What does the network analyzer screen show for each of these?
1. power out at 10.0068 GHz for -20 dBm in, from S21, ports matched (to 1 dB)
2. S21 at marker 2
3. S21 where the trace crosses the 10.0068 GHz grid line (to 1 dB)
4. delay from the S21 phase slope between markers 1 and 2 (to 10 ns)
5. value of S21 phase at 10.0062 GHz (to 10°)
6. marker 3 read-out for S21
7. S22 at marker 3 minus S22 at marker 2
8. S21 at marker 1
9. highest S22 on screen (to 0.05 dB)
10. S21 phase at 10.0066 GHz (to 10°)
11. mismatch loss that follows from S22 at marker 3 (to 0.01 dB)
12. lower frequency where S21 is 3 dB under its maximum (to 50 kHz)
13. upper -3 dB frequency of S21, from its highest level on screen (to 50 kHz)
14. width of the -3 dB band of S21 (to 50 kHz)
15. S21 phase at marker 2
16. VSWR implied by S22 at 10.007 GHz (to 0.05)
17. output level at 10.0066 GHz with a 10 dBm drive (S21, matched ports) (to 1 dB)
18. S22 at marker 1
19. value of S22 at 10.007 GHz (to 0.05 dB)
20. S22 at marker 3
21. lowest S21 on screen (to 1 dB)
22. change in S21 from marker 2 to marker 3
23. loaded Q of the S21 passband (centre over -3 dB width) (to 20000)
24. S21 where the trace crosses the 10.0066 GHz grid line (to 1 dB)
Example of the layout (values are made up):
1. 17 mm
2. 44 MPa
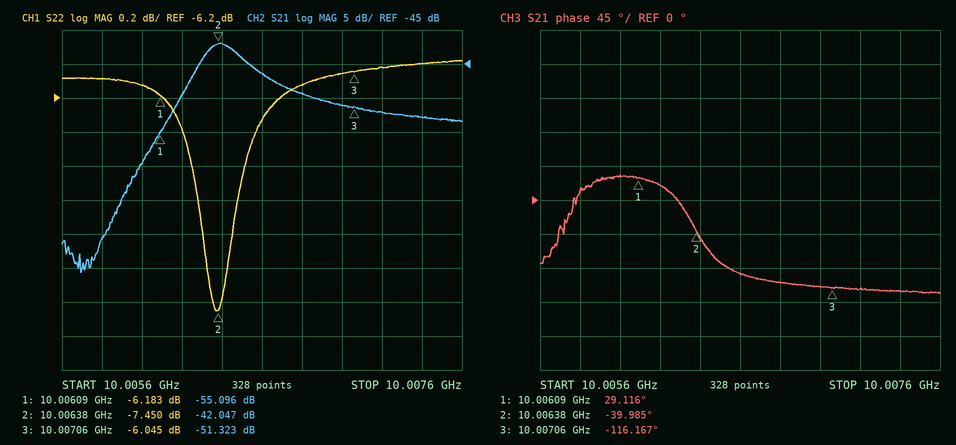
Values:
1. -69 dBm
2. -42.047 dB
3. -49 dB
4. 660 ns
5. 20°
6. -51.323 dB
7. 1.405 dB
8. -55.096 dB
9. -6.00 dB
10. -100°
11. 1.24 dB
12. 10.00630 GHz
13. 10.00655 GHz
14. 250 kHz
15. -39.985°
16. 3.00
17. -36 dBm
18. -6.183 dB
19. -6.05 dB
20. -6.045 dB
21. -76 dB
22. -9.276 dB
23. 40000
24. -46 dB
